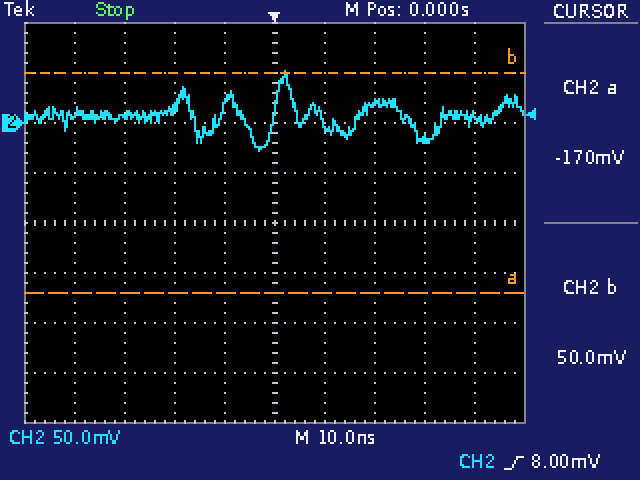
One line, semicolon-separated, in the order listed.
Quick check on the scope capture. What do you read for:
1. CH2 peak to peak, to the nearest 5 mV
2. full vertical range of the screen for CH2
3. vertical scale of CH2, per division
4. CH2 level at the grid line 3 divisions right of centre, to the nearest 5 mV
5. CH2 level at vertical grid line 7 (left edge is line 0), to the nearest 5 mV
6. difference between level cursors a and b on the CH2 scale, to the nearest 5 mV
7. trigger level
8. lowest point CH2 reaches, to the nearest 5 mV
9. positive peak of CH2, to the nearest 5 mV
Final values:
80 mV; 400 mV; 50 mV; -15 mV; 20 mV; 220 mV; 8.00 mV; -30 mV; 50 mV
